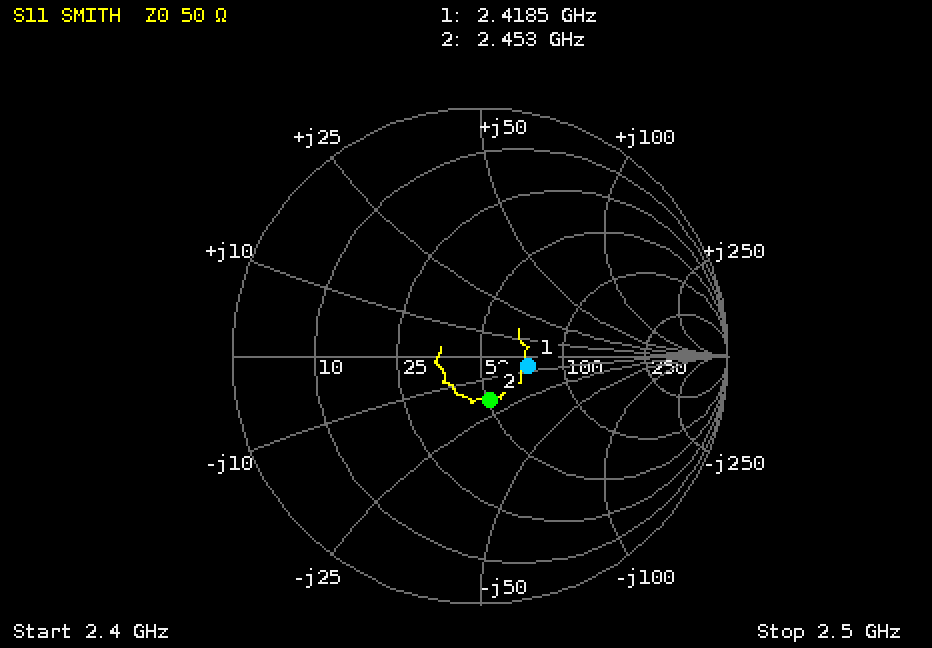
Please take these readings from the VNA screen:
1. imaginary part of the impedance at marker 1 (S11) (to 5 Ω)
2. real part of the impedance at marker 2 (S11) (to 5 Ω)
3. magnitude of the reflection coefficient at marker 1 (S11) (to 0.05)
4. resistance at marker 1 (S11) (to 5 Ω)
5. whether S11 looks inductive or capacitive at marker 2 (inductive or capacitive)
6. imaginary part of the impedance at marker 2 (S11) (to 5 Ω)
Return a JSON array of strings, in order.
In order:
["-5 Ω", "50 Ω", "0.20", "75 Ω", "capacitive", "-20 Ω"]
